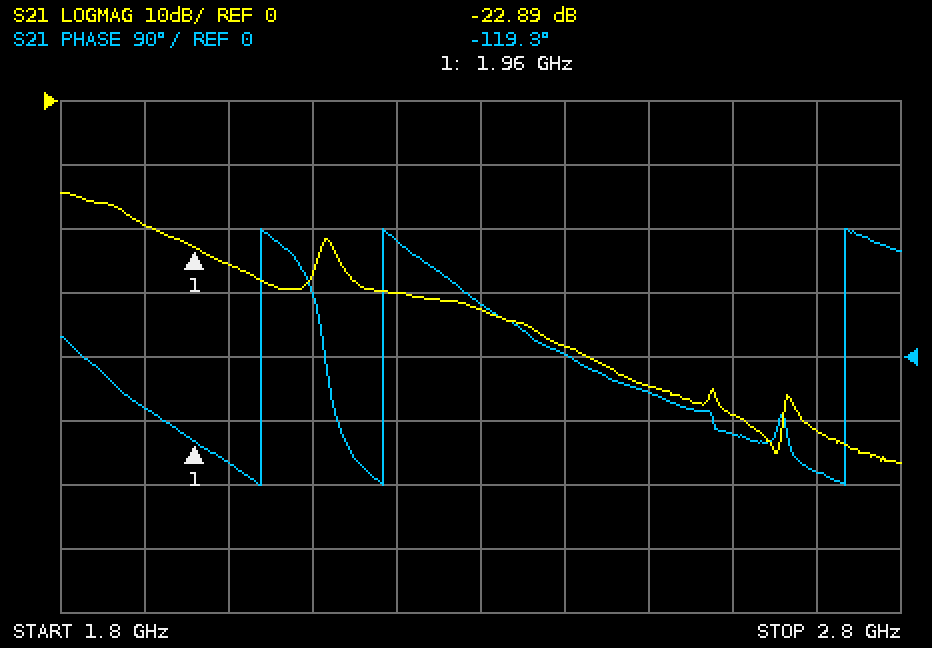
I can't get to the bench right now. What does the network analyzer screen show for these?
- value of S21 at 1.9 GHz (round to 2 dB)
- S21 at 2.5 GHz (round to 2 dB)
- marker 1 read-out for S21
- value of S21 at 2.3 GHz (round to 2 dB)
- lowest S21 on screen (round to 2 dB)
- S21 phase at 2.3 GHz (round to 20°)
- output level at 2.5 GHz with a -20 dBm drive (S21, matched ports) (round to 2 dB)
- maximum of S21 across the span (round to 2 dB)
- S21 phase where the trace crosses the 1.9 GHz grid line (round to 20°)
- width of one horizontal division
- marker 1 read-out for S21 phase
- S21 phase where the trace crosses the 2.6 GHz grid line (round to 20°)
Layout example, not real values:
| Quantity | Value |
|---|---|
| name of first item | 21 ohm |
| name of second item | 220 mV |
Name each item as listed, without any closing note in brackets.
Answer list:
| Quantity | Value |
|---|---|
| value of S21 at 1.9 GHz | -20 dB |
| S21 at 2.5 GHz | -44 dB |
| marker 1 read-out for S21 | -22.89 dB |
| value of S21 at 2.3 GHz | -32 dB |
| lowest S21 on screen | -56 dB |
| S21 phase at 2.3 GHz | 80° |
| output level at 2.5 GHz with a -20 dBm drive (S21, matched ports) | -64 dBm |
| maximum of S21 across the span | -14 dB |
| S21 phase where the trace crosses the 1.9 GHz grid line | -80° |
| width of one horizontal division | 100 MHz |
| marker 1 read-out for S21 phase | -119.3° |
| S21 phase where the trace crosses the 2.6 GHz grid line | -100° |
